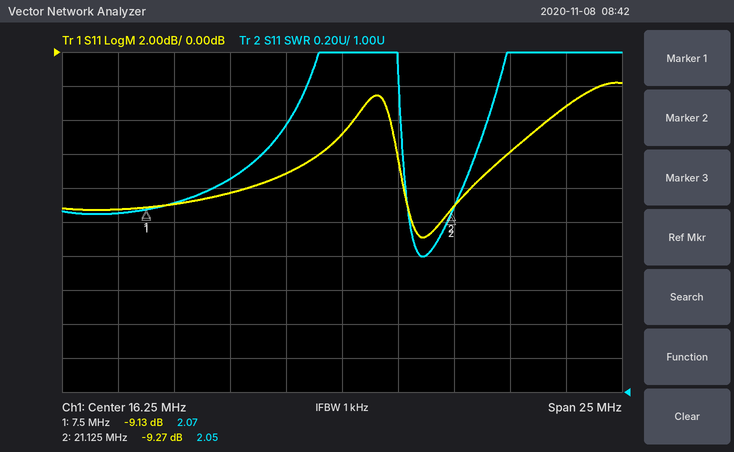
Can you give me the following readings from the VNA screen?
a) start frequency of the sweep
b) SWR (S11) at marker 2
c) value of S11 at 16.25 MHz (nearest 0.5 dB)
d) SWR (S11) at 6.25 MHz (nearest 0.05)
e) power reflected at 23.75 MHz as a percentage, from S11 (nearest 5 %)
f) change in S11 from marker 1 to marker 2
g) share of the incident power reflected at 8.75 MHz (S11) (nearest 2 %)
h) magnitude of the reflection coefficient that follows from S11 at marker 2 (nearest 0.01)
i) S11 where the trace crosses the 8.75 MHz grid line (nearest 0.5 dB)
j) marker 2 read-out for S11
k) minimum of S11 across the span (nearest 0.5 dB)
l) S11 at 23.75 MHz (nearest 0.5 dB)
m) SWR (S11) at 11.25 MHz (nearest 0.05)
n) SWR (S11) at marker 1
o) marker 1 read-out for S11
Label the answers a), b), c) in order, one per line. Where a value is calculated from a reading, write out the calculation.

a) 3.75 MHz
b) 2.05
c) -5.0 dB
d) 2.05
e) 10^(-6/10) ≈ 25 %
f) -9.27 − (-9.13) = -0.14 dB
g) 10^(-9/10) ≈ 12.6 %, so 12 % to the nearest 2 %
h) 10^(-9.27/20) ≈ 0.34
i) -9.0 dB
j) -9.27 dB
k) -11.0 dB
l) -6.0 dB
m) 2.25
n) 2.07
o) -9.13 dB
